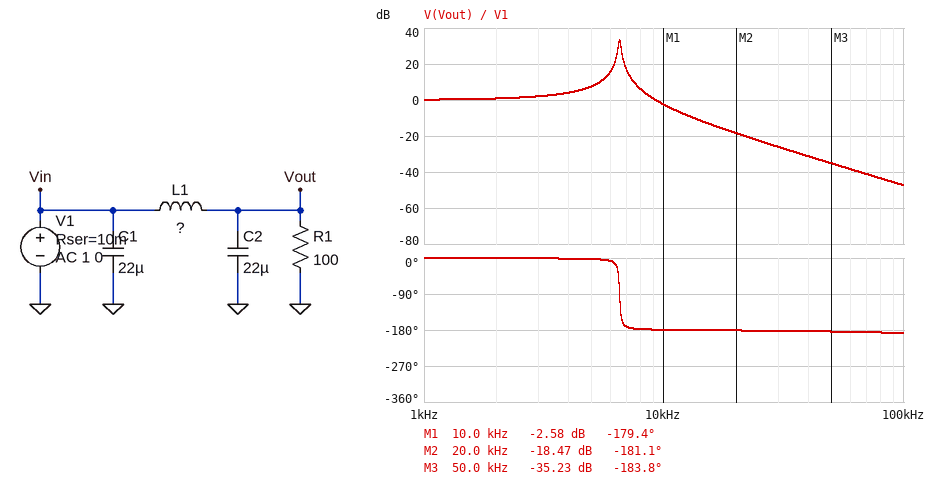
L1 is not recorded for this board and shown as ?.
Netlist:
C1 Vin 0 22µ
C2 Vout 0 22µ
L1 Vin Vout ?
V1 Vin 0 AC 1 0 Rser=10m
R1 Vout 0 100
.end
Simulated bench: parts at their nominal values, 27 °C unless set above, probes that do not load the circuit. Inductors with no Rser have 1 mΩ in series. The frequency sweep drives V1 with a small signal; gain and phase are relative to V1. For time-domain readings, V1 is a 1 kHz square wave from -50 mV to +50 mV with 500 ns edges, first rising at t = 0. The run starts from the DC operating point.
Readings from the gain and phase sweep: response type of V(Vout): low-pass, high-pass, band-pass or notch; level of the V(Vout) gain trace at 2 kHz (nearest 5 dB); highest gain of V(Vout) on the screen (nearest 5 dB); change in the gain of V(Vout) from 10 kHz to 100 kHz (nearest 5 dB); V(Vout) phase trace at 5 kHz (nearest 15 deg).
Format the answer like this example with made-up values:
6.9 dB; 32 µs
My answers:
low-pass; 0 dB; 35 dB; -45 dB; 0 deg
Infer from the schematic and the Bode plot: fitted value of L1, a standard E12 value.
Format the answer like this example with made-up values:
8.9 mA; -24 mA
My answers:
27 µH
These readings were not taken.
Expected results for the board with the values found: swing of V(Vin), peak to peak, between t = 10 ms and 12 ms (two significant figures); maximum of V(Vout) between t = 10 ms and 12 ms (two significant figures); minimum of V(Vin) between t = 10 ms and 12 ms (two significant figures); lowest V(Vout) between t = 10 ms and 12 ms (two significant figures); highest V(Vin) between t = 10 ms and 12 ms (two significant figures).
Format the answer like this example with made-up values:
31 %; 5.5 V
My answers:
100 mV; 130 mV; -51 mV; -130 mV; 51 mV
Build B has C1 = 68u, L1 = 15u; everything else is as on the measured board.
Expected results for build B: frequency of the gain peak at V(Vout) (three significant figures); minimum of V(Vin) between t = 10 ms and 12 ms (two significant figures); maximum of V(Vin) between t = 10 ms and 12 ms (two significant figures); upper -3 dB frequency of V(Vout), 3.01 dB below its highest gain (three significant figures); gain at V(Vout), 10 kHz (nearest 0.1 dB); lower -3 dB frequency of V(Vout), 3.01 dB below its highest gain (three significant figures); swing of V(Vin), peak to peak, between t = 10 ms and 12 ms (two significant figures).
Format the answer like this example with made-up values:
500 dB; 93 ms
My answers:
8.76 kHz; -52 mV; 52 mV; 8.86 kHz; 10.4 dB; 8.67 kHz; 100 mV
